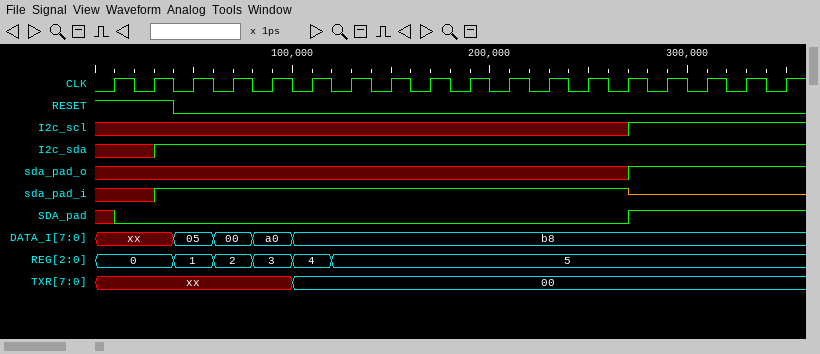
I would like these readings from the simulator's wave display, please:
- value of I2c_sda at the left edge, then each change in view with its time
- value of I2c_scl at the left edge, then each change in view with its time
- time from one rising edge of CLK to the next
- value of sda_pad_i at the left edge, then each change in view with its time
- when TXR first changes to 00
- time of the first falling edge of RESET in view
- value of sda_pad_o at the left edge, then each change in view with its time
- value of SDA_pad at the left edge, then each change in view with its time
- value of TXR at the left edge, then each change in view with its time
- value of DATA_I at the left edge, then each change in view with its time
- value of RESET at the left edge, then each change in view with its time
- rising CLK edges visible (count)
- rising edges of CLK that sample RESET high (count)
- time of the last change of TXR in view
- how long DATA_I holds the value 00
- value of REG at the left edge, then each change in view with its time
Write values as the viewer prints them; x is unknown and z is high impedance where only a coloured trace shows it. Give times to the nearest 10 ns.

x, 1 at 30 ns
x, 1 at 270 ns
20 ns
x, 1 at 30 ns, z at 270 ns
100 ns
40 ns
x, 1 at 270 ns
x, 0 at 10 ns, 1 at 270 ns
xx, 00 at 100 ns
xx, 05 at 40 ns, 00 at 60 ns, a0 at 80 ns, b8 at 100 ns
1, 0 at 40 ns
18
2
100 ns
20 ns
0, 1 at 40 ns, 2 at 60 ns, 3 at 80 ns, 4 at 100 ns, 5 at 120 ns
